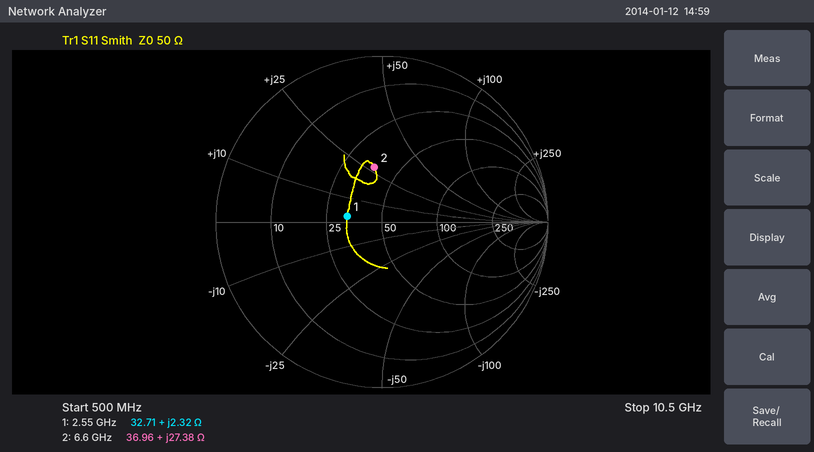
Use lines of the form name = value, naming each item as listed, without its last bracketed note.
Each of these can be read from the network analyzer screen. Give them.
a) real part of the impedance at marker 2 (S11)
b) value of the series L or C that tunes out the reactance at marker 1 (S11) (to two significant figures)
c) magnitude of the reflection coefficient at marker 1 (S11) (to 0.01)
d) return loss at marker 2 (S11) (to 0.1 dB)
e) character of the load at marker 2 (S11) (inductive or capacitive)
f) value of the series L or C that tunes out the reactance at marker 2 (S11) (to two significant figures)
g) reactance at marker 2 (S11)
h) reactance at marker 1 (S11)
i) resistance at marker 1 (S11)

real part of the impedance at marker 2 = 36.96 Ω
value of the series L or C that tunes out the reactance at marker 1 (S11) = 27 pF
magnitude of the reflection coefficient at marker 1 (S11) = 0.21
return loss at marker 2 (S11) = 9.6 dB
character of the load at marker 2 (S11) = inductive
value of the series L or C that tunes out the reactance at marker 2 (S11) = 880 fF
reactance at marker 2 = +27.38 Ω
reactance at marker 1 = +2.32 Ω
resistance at marker 1 = 32.71 Ω
